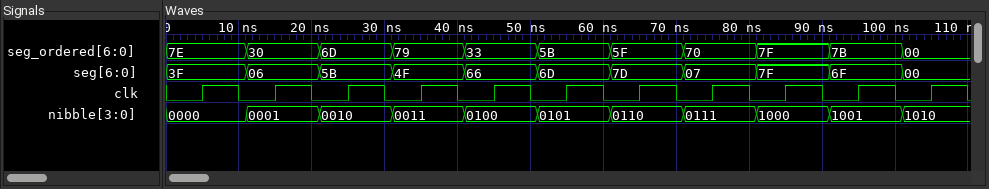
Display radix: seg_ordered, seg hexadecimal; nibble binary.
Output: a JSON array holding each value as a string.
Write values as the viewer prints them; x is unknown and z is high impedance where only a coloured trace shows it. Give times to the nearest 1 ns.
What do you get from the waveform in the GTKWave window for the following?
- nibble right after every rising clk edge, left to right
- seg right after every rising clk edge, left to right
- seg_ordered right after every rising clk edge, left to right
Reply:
["0000, 0001, 0010, 0011, 0100, 0101, 0110, 0111, 1000, 1001, 1010", "3F, 06, 5B, 4F, 66, 6D, 7D, 07, 7F, 6F, 00", "7E, 30, 6D, 79, 33, 5B, 5F, 70, 7F, 7B, 00"]
